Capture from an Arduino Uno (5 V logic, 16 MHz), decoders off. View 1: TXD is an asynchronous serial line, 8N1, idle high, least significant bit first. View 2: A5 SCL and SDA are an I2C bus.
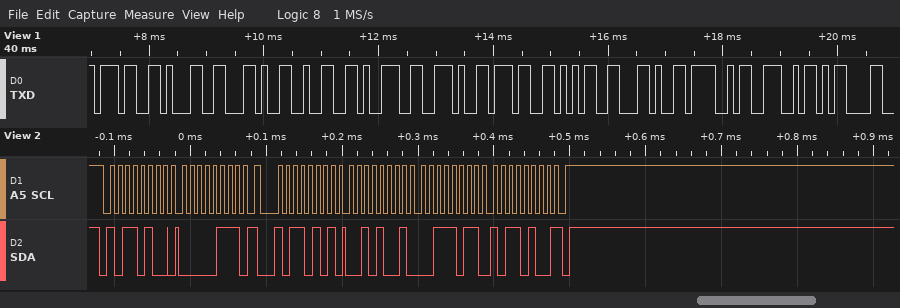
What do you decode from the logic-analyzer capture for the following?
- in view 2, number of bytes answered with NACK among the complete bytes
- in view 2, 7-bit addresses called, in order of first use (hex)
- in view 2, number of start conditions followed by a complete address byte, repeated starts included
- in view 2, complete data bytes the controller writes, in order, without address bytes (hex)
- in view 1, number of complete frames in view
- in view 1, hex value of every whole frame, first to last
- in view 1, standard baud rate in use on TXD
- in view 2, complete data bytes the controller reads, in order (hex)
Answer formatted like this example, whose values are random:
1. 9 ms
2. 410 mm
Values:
1. 1
2. 0x5A
3. 2
4. 07
5. 12
6. 0x37 0x31 0x2C 0x32 0x39 0x2E 0x37 0x35 0x2C 0x4F 0x4E 0x0D
7. 9600 baud
8. 29 3B B4
